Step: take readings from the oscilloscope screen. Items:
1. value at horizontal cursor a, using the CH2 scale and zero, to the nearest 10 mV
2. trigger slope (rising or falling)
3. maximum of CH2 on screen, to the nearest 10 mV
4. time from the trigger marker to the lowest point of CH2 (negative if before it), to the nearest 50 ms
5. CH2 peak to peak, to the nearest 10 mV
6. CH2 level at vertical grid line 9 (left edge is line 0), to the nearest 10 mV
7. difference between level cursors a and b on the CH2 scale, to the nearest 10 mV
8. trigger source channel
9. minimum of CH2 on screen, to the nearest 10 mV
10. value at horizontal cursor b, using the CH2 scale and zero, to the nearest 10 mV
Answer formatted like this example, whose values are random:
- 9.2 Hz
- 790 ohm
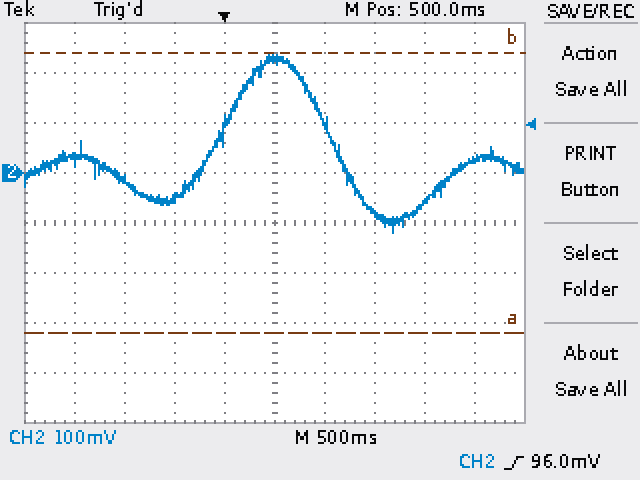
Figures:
- -320 mV
- rising
- 240 mV
- +1.70 s
- 360 mV
- 30 mV
- 560 mV
- CH2
- -120 mV
- 240 mV
